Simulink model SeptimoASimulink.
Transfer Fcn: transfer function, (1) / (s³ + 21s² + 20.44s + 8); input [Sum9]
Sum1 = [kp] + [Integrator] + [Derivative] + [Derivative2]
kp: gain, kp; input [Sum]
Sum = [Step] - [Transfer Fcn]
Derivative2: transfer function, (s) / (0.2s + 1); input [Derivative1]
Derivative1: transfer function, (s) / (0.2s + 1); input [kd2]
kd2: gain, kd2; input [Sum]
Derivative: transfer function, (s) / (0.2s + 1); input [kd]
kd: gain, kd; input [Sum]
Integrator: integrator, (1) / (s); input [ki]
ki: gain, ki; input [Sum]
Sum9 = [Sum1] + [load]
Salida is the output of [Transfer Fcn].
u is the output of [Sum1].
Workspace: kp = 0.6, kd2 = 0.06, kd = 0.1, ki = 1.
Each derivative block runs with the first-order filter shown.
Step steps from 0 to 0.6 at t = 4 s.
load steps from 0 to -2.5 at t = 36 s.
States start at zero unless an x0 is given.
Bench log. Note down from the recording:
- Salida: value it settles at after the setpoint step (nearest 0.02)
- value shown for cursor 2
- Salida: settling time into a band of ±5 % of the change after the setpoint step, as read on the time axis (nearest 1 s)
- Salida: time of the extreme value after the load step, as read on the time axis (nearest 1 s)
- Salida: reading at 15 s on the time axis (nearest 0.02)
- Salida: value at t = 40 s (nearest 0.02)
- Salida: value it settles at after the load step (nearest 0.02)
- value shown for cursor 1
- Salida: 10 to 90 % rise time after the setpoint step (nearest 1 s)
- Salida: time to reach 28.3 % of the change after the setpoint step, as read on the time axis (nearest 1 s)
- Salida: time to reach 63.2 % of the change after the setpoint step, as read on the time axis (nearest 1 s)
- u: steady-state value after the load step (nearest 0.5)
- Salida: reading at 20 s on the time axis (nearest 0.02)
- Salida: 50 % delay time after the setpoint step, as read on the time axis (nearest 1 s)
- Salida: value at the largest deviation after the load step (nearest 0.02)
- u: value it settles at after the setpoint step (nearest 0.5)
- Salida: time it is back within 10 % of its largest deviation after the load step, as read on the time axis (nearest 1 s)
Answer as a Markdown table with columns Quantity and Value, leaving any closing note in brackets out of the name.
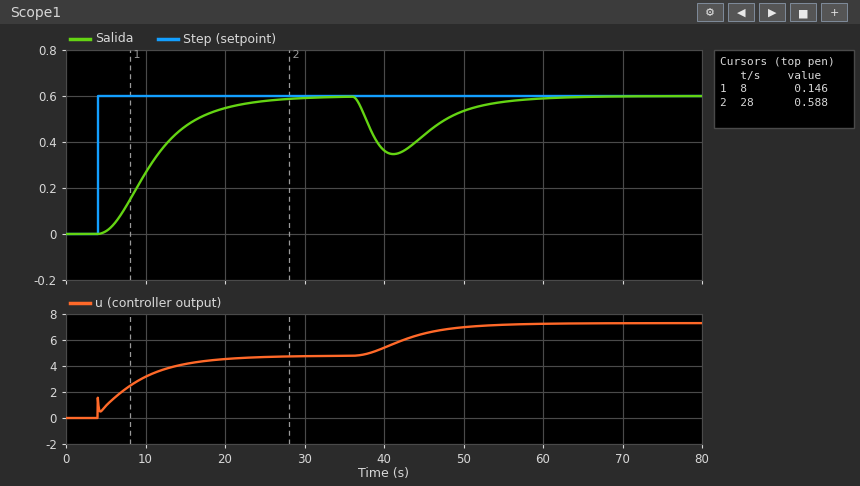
| Quantity | Value |
|---|---|
| Salida: value it settles at after the setpoint step | 0.60 |
| value shown for cursor 2 | 0.588 |
| Salida: settling time into a band of ±5 % of the change after the setpoint step, as read on the time axis | 23 s |
| Salida: time of the extreme value after the load step, as read on the time axis | 41 s |
| Salida: reading at 15 s on the time axis | 0.46 |
| Salida: value at t = 40 s | 0.36 |
| Salida: value it settles at after the load step | 0.60 |
| value shown for cursor 1 | 0.146 |
| Salida: 10 to 90 % rise time after the setpoint step | 13 s |
| Salida: time to reach 28.3 % of the change after the setpoint step, as read on the time axis | 8 s |
| Salida: time to reach 63.2 % of the change after the setpoint step, as read on the time axis | 12 s |
| u: steady-state value after the load step | 7.5 |
| Salida: reading at 20 s on the time axis | 0.54 |
| Salida: 50 % delay time after the setpoint step, as read on the time axis | 11 s |
| Salida: value at the largest deviation after the load step | 0.34 |
| u: value it settles at after the setpoint step | 5.0 |
| Salida: time it is back within 10 % of its largest deviation after the load step, as read on the time axis | 55 s |
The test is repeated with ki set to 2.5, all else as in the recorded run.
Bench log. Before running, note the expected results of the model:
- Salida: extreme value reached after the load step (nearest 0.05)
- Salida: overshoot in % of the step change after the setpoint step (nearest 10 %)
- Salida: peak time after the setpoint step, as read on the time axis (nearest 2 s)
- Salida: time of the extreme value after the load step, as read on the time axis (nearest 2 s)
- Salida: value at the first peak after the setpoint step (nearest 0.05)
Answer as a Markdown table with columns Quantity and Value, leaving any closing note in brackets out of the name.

| Quantity | Value |
|---|---|
| Salida: extreme value reached after the load step | 0.40 |
| Salida: overshoot in % of the step change after the setpoint step | 20 % |
| Salida: peak time after the setpoint step, as read on the time axis | 14 s |
| Salida: time of the extreme value after the load step, as read on the time axis | 40 s |
| Salida: value at the first peak after the setpoint step | 0.70 |
